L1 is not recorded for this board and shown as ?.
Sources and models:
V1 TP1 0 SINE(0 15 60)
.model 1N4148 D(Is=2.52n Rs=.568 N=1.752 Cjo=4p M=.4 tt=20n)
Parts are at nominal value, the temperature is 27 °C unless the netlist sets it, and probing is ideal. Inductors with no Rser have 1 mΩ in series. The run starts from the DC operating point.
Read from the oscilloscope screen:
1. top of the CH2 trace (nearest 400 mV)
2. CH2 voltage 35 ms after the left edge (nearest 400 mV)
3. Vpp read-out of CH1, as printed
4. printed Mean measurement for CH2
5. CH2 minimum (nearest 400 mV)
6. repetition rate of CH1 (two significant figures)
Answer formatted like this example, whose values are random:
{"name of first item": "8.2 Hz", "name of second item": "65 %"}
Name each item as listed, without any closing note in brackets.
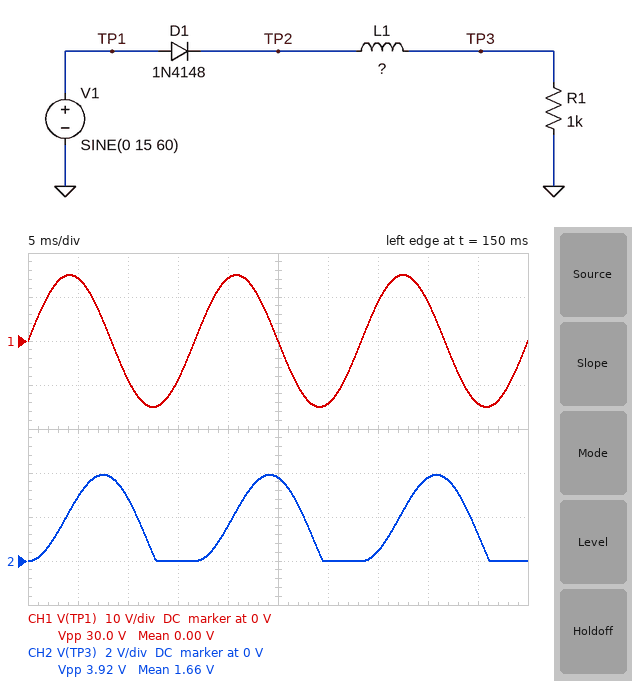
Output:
{"top of the CH2 trace": "4.0 V", "CH2 voltage 35 ms after the left edge": "400 mV", "Vpp read-out of CH1, as printed": "30.0 V", "printed Mean measurement for CH2": "1.66 V", "CH2 minimum": "0 V", "repetition rate of CH1": "60 Hz"}
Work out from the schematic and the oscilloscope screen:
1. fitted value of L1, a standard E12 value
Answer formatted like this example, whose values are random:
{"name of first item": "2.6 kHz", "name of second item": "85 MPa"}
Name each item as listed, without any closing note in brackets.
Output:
{"fitted value of L1, a standard E12 value": "15 H"}
